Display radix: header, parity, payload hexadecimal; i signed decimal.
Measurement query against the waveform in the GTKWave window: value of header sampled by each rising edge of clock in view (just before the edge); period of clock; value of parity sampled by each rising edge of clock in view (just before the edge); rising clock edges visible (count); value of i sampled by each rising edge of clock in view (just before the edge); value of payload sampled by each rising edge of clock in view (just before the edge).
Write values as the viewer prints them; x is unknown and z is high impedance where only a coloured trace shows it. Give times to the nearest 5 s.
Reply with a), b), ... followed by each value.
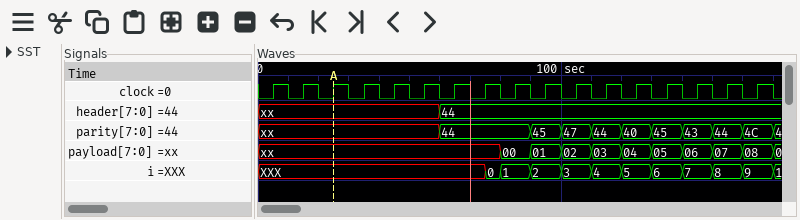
a) xx, xx, xx, xx, xx, xx, 44, 44, 44, 44, 44, 44, 44, 44, 44, 44, 44
b) 10 s
c) xx, xx, xx, xx, xx, xx, 44, 44, 44, 45, 47, 44, 40, 45, 43, 44, 4C
d) 17
e) XXX, XXX, XXX, XXX, XXX, XXX, XXX, XXX, 1, 2, 3, 4, 5, 6, 7, 8, 9
f) xx, xx, xx, xx, xx, xx, xx, xx, 00, 01, 02, 03, 04, 05, 06, 07, 08
